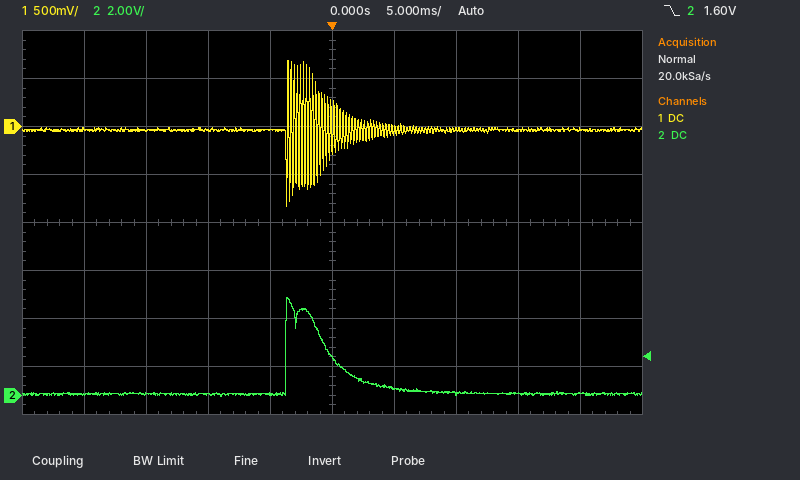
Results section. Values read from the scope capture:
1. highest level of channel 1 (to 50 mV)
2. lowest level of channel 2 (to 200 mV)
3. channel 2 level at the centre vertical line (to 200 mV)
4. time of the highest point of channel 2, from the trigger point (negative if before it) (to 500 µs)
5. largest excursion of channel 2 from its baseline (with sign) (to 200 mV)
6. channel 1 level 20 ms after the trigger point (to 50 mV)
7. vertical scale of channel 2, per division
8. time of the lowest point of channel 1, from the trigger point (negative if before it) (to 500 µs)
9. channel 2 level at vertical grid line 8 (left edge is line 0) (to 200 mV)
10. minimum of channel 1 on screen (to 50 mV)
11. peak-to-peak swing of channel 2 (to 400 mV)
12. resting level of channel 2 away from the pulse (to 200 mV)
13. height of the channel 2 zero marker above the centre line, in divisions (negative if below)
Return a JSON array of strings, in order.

["700 mV", "0.0 V", "1.6 V", "-3.5 ms", "+4.0 V", "-50 mV", "2 V", "-3.5 ms", "0.0 V", "-850 mV", "4.0 V", "0.0 V", "-3.6 div"]
